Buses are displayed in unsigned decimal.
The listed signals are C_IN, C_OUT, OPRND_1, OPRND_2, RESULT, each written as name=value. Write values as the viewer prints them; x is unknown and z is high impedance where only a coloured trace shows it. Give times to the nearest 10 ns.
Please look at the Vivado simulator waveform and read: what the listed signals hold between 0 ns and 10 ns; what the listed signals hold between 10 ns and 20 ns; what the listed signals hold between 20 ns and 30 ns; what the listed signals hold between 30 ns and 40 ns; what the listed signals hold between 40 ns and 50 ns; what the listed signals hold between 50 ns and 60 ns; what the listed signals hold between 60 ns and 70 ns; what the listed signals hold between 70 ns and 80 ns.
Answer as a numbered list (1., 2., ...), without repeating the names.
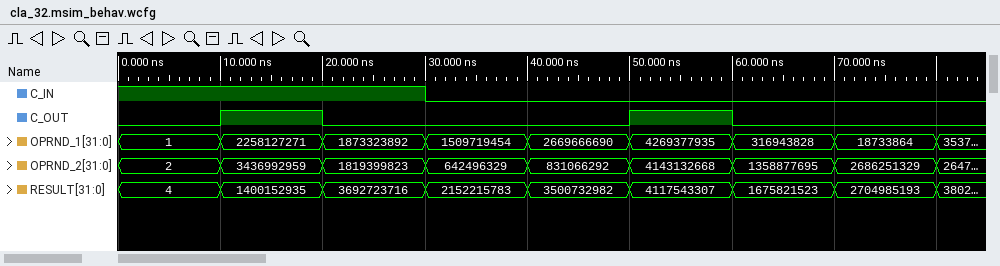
1. C_IN=1, C_OUT=0, OPRND_1=1, OPRND_2=2, RESULT=4
2. C_IN=1, C_OUT=1, OPRND_1=2258127271, OPRND_2=3436992959, RESULT=1400152935
3. C_IN=1, C_OUT=0, OPRND_1=1873323892, OPRND_2=1819399823, RESULT=3692723716
4. C_IN=0, C_OUT=0, OPRND_1=1509719454, OPRND_2=642496329, RESULT=2152215783
5. C_IN=0, C_OUT=0, OPRND_1=2669666690, OPRND_2=831066292, RESULT=3500732982
6. C_IN=0, C_OUT=1, OPRND_1=4269377935, OPRND_2=4143132668, RESULT=4117543307
7. C_IN=0, C_OUT=0, OPRND_1=316943828, OPRND_2=1358877695, RESULT=1675821523
8. C_IN=0, C_OUT=0, OPRND_1=18733864, OPRND_2=2686251329, RESULT=2704985193
